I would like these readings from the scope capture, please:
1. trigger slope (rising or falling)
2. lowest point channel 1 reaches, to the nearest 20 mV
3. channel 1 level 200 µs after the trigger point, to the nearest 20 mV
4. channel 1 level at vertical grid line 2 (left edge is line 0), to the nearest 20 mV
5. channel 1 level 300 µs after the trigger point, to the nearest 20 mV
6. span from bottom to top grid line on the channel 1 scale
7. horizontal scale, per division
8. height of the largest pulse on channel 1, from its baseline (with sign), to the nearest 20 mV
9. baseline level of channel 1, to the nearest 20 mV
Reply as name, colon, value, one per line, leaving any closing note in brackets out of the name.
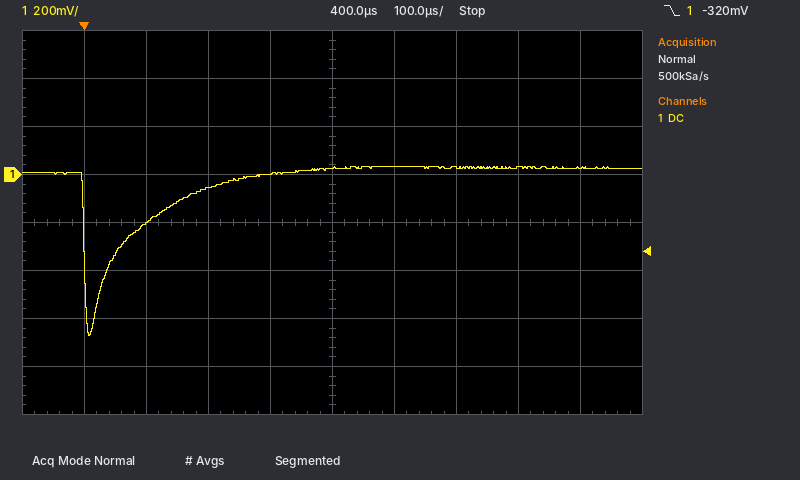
trigger slope: falling
lowest point channel 1 reaches, to the nearest 20 mV: -680 mV
channel 1 level 200 µs after the trigger point, to the nearest 20 mV: -60 mV
channel 1 level at vertical grid line 2 (left edge is line 0), to the nearest 20 mV: -200 mV
channel 1 level 300 µs after the trigger point, to the nearest 20 mV: 0 mV
span from bottom to top grid line on the channel 1 scale: 1.6 V
horizontal scale, per division: 100 µs
height of the largest pulse on channel 1, from its baseline (with sign), to the nearest 20 mV: -700 mV
baseline level of channel 1, to the nearest 20 mV: 20 mV
